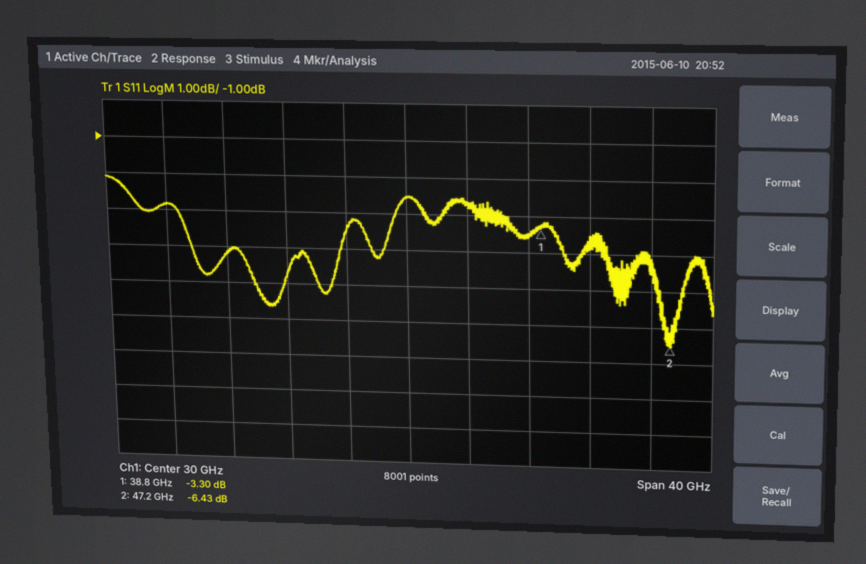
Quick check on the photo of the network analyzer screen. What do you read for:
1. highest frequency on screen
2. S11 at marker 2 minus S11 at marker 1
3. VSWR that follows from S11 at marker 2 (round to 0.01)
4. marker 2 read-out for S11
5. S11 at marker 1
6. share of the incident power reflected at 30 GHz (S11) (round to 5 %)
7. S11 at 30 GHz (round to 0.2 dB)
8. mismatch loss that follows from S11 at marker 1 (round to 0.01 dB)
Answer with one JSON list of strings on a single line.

["50 GHz", "-3.13 dB", "2.82", "-6.43 dB", "-3.30 dB", "55 %", "-2.6 dB", "2.74 dB"]
